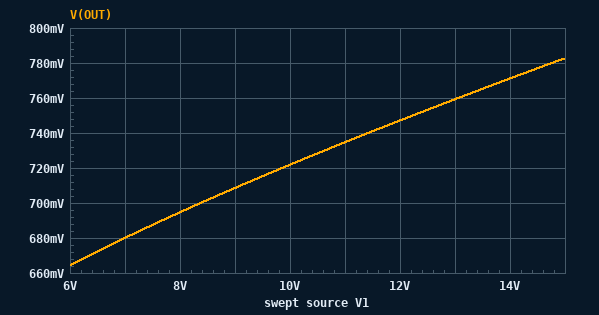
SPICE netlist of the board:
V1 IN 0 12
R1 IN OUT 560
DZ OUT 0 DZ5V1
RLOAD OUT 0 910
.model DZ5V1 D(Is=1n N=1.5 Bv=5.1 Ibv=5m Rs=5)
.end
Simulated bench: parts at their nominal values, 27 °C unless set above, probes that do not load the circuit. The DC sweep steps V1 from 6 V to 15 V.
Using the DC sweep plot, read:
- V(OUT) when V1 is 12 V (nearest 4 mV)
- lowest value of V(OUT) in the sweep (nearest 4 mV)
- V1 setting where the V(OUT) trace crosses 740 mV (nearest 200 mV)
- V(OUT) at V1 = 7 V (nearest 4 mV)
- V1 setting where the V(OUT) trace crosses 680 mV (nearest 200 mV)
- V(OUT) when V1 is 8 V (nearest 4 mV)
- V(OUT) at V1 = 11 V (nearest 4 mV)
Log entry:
748 mV
664 mV
11.4 V
680 mV
7.0 V
696 mV
736 mV
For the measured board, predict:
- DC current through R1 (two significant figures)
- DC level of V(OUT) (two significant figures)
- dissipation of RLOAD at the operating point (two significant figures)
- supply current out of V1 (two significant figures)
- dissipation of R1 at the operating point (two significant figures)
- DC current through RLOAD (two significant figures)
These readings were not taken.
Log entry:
20 mA
750 mV
610 µW
20 mA
230 mW
820 µA
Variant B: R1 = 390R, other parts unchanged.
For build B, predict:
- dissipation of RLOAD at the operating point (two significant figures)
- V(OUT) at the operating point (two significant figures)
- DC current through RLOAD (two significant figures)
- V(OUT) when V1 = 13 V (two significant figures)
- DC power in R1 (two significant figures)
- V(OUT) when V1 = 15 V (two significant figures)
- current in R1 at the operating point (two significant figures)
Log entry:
710 µW
800 mV
880 µA
820 mV
320 mW
850 mV
29 mA
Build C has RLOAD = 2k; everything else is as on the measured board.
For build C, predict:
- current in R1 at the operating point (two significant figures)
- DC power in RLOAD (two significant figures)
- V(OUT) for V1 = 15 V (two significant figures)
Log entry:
20 mA
280 µW
790 mV
